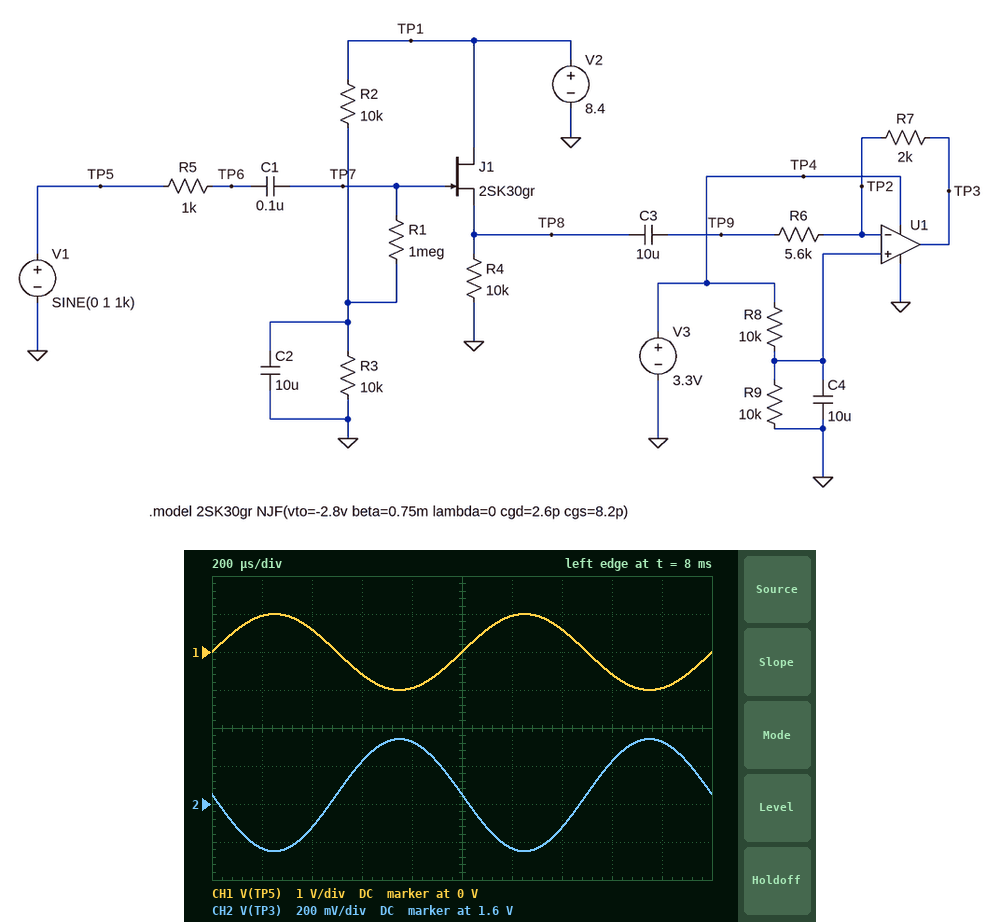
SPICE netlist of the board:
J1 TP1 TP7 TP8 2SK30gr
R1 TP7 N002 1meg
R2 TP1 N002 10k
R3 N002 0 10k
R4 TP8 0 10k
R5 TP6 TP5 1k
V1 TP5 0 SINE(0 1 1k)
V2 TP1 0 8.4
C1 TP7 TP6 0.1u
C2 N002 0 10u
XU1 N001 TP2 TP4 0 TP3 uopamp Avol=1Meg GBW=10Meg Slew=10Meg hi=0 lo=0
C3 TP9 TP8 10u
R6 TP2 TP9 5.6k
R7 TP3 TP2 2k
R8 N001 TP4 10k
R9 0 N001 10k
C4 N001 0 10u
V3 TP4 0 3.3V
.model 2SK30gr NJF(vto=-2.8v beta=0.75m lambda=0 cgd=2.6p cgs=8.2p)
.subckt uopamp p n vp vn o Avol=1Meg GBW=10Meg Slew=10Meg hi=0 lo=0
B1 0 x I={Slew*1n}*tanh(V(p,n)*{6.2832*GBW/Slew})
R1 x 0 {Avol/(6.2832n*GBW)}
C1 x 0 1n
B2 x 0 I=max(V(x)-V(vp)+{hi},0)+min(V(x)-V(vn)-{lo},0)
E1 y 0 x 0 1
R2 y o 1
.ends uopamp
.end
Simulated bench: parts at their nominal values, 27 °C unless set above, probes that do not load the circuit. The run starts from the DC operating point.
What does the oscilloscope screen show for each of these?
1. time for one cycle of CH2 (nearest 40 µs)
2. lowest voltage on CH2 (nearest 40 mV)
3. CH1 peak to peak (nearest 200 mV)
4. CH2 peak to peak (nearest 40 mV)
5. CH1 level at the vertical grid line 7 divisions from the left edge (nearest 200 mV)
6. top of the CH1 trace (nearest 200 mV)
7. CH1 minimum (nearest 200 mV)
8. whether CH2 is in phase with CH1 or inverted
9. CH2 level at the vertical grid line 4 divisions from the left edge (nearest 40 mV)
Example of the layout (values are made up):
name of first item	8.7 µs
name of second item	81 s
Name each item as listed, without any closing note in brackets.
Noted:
time for one cycle of CH2	1.00 ms
lowest voltage on CH2	1.36 V
CH1 peak to peak	2.0 V
CH2 peak to peak	600 mV
CH1 level at the vertical grid line 7 divisions from the left edge	600 mV
top of the CH1 trace	1.0 V
CH1 minimum	-1.0 V
whether CH2 is in phase with CH1 or inverted	inverted
CH2 level at the vertical grid line 4 divisions from the left edge	1.92 V
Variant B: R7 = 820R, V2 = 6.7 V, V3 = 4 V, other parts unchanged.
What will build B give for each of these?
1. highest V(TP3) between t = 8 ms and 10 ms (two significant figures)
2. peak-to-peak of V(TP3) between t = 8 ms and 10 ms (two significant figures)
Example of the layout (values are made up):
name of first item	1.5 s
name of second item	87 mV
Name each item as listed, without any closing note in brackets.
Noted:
highest V(TP3) between t = 8 ms and 10 ms	2.1 V
peak-to-peak of V(TP3) between t = 8 ms and 10 ms	230 mV
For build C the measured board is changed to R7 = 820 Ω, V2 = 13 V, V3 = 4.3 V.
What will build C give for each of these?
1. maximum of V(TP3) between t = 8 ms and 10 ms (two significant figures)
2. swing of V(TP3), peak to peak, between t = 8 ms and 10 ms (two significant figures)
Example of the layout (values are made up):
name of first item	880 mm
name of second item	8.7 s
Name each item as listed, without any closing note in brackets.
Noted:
maximum of V(TP3) between t = 8 ms and 10 ms	2.3 V
swing of V(TP3), peak to peak, between t = 8 ms and 10 ms	250 mV
